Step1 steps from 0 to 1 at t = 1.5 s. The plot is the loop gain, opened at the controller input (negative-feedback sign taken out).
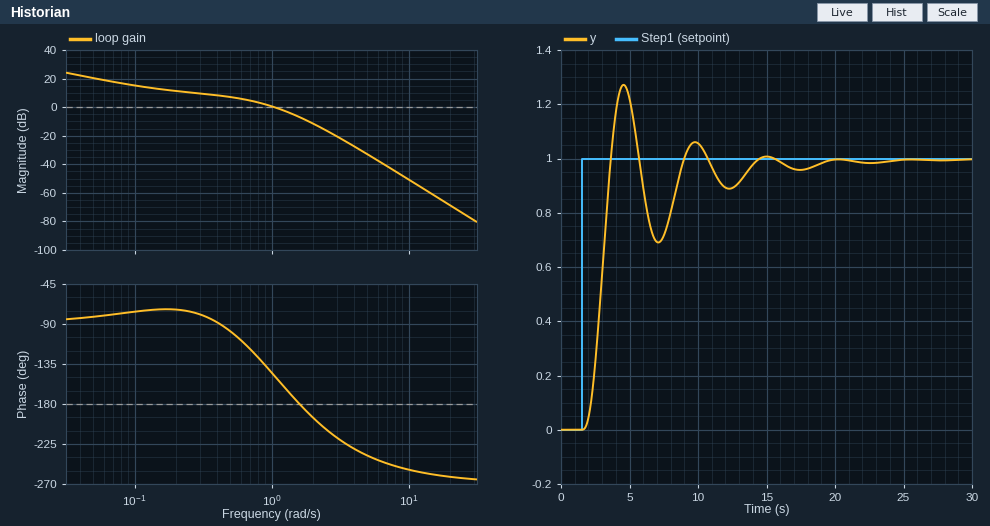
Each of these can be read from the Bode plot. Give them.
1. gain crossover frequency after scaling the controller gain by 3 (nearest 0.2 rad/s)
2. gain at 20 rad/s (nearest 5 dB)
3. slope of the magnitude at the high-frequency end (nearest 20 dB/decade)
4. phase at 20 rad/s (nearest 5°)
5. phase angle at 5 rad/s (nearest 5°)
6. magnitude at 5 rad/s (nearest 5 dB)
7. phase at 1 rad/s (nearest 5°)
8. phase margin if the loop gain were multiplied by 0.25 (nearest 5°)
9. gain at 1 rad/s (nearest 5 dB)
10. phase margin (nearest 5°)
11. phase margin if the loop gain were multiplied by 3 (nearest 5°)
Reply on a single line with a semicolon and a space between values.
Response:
1.8 rad/s; -70 dB; -60 dB/decade; -260°; -240°; -35 dB; -145°; 105°; 0 dB; 30°; -10°
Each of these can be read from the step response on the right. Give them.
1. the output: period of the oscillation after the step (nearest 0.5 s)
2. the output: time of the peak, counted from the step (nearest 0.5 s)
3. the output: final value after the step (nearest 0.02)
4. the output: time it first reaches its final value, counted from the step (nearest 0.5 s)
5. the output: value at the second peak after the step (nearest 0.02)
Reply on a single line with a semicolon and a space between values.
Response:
5.0 s; 3.0 s; 1.00; 2.0 s; 1.06
